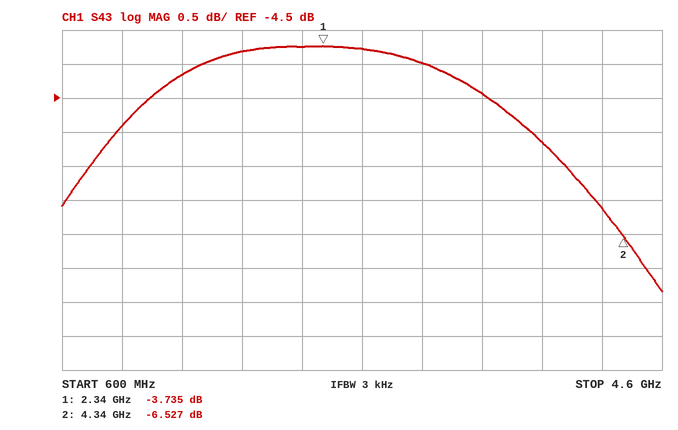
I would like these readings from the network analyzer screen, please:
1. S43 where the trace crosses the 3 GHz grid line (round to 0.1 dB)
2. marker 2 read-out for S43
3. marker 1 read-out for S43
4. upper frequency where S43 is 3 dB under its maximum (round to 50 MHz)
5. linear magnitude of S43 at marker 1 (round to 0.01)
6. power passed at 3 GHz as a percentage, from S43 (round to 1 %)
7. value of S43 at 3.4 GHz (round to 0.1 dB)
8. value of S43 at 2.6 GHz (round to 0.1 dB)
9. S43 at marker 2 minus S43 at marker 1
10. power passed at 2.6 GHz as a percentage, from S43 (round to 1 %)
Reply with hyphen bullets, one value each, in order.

- -4.0 dB
- -6.527 dB
- -3.735 dB
- 4.40 GHz
- 0.65
- 40 %
- -4.4 dB
- -3.8 dB
- -2.792 dB
- 42 %
